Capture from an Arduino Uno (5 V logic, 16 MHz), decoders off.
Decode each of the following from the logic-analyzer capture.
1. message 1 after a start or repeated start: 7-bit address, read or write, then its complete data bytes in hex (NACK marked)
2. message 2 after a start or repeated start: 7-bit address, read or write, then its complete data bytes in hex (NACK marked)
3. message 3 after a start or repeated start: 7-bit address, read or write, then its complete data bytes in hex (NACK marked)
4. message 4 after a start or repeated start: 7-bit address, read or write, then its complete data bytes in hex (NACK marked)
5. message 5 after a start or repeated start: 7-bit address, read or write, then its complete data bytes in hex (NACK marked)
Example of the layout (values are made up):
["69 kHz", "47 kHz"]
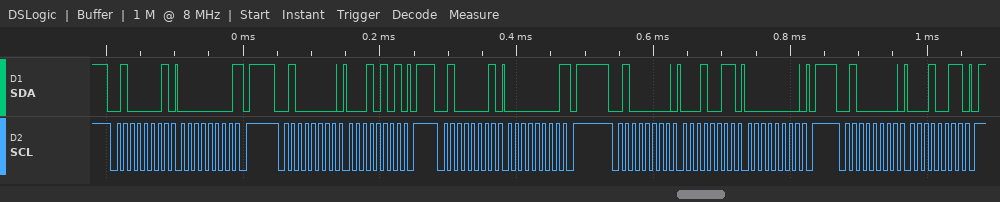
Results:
["0x20 read: 00 NACK", "0x20 write: 15", "0x20 read: 00 NACK", "0x20 write: 13 00", "0x20 write: 13"]
